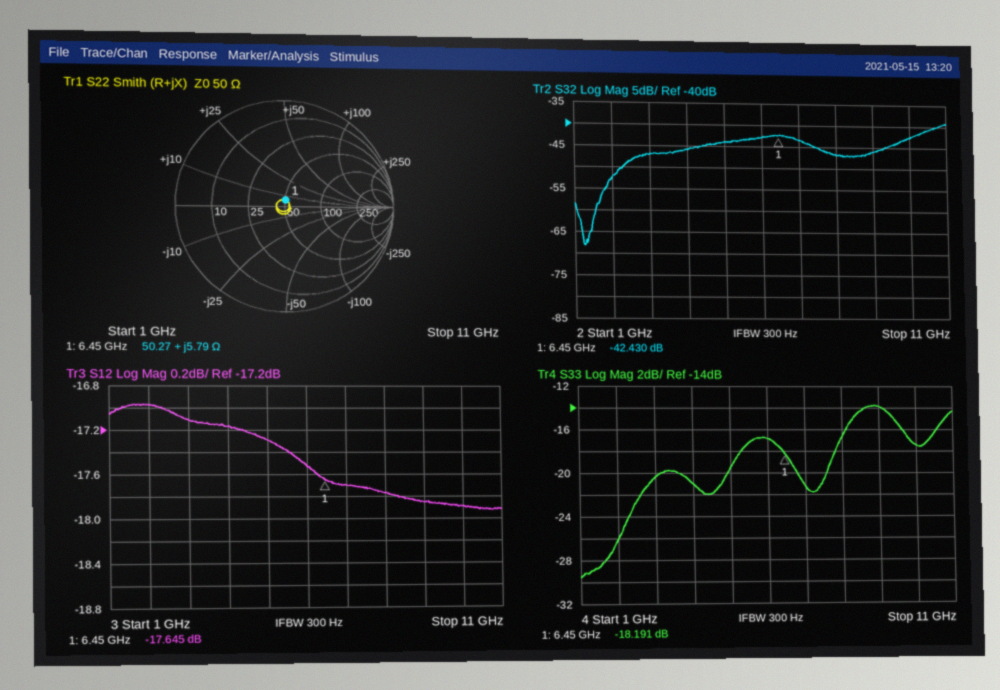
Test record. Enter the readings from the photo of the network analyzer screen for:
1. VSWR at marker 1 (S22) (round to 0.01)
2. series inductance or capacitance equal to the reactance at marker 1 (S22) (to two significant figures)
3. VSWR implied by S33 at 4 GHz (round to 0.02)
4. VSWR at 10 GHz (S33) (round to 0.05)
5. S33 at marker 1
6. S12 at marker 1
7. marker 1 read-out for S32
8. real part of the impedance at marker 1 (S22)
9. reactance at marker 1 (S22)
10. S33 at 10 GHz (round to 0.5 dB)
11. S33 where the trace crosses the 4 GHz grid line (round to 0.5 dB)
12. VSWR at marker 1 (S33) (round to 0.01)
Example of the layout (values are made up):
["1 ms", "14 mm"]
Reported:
["1.12", "140 pH", "1.20", "1.30", "-18.191 dB", "-17.645 dB", "-42.430 dB", "50.27 Ω", "+5.79 Ω", "-17.5 dB", "-21.0 dB", "1.28"]
